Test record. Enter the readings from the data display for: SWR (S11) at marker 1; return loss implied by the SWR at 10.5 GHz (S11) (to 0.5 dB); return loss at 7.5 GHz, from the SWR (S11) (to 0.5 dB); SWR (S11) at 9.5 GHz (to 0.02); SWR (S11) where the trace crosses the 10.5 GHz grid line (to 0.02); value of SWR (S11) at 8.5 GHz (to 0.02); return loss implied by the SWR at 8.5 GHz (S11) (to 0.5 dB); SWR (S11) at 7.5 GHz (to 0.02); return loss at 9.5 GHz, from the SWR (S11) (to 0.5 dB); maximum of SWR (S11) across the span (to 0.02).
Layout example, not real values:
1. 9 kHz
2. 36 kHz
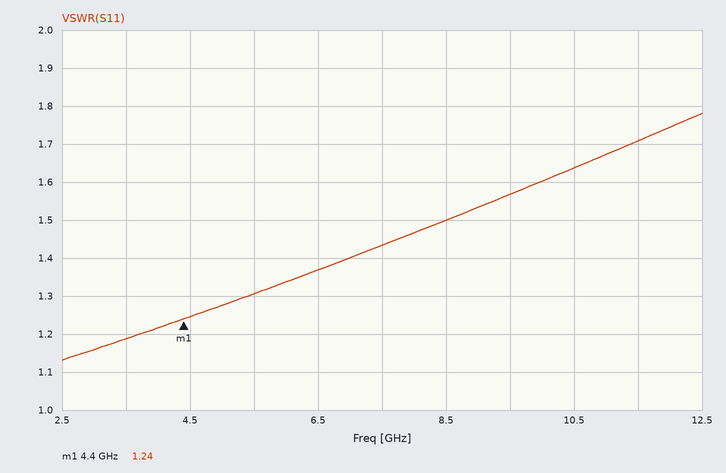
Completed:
1. 1.24
2. 12.5 dB
3. 15.0 dB
4. 1.56
5. 1.64
6. 1.50
7. 14.0 dB
8. 1.44
9. 13.0 dB
10. 1.78
